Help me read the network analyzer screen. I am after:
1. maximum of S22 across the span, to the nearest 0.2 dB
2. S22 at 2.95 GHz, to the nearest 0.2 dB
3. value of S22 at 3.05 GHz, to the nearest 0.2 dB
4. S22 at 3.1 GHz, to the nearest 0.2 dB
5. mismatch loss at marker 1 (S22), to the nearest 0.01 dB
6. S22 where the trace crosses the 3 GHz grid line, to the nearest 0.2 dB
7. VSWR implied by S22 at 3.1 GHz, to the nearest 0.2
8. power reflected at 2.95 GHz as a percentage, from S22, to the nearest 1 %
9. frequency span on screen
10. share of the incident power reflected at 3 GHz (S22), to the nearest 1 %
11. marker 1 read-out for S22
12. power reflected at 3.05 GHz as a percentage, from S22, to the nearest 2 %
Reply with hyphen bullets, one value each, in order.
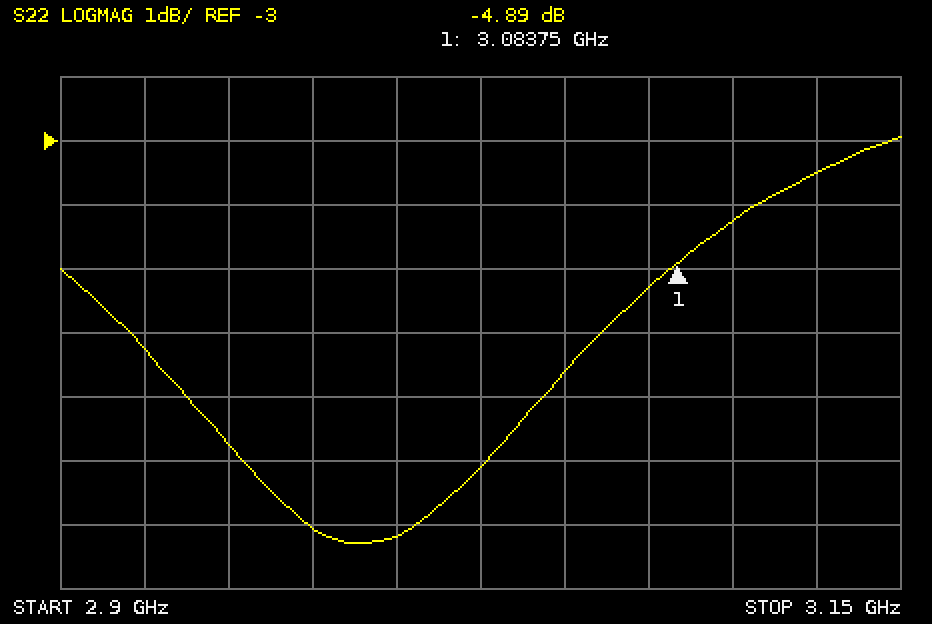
- -3.0 dB
- -7.8 dB
- -6.6 dB
- -4.2 dB
- 1.70 dB
- -9.2 dB
- 4.2
- 17 %
- 250 MHz
- 12 %
- -4.89 dB
- 22 %
